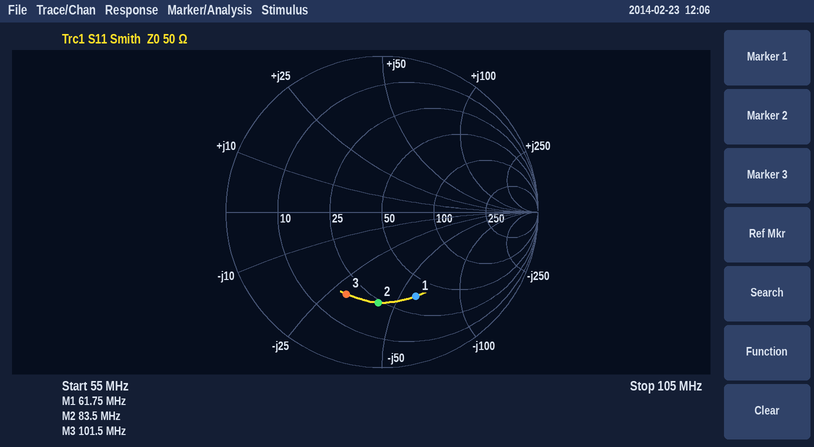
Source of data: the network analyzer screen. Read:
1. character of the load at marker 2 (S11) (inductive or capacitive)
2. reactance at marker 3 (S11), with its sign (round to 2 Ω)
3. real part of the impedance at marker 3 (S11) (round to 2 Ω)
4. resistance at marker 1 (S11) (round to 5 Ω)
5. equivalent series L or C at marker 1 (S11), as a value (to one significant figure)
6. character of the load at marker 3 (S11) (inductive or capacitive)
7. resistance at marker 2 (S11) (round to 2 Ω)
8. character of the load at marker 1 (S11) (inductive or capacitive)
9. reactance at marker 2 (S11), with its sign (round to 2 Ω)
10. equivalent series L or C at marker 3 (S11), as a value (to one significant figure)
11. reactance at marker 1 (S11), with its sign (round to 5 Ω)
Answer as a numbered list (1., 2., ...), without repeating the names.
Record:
1. capacitive
2. -30 Ω
3. 18 Ω
4. 35 Ω
5. 40 pF
6. capacitive
7. 24 Ω
8. capacitive
9. -42 Ω
10. 50 pF
11. -60 Ω
